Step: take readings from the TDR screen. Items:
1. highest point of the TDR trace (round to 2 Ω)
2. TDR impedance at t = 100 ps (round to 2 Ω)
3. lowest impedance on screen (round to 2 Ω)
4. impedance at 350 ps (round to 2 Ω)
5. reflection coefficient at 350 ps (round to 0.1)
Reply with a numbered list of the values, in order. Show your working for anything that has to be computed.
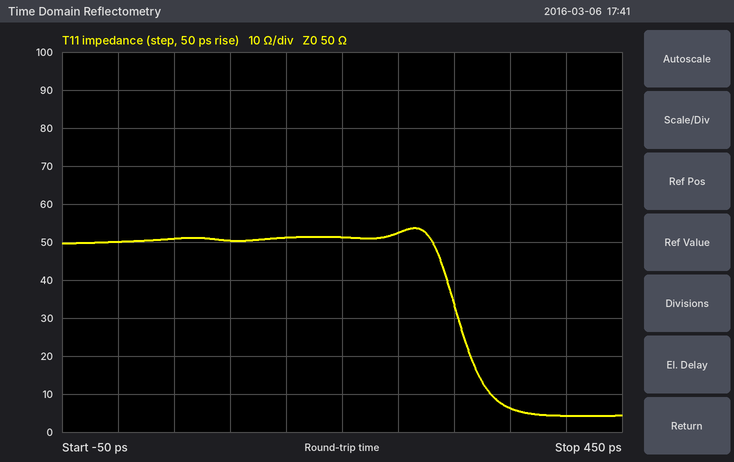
1. 54 Ω
2. 50 Ω
3. 4 Ω
4. 6 Ω
5. (6 − 50)/(6 + 50) ≈ -0.8
